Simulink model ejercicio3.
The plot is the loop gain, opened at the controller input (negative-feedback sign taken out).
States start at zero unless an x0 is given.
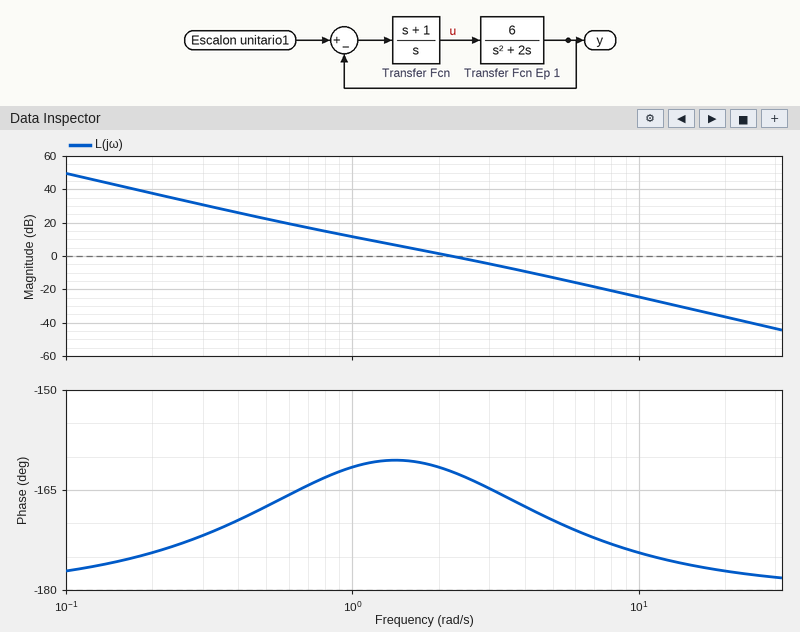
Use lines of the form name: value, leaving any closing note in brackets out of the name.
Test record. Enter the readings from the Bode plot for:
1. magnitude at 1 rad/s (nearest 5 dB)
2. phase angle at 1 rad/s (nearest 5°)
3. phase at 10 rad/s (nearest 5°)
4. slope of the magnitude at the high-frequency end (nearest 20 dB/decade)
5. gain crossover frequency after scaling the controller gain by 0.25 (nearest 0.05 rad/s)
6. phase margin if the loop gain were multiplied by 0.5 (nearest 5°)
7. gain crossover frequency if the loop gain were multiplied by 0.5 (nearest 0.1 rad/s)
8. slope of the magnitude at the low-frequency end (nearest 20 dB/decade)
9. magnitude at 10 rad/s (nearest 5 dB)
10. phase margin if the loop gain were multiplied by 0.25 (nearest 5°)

magnitude at 1 rad/s: 10 dB
phase angle at 1 rad/s: -160°
phase at 10 rad/s: -175°
slope of the magnitude at the high-frequency end: -40 dB/decade
gain crossover frequency after scaling the controller gain by 0.25: 0.95 rad/s
phase margin if the loop gain were multiplied by 0.5: 20°
gain crossover frequency if the loop gain were multiplied by 0.5: 1.5 rad/s
slope of the magnitude at the low-frequency end: -40 dB/decade
magnitude at 10 rad/s: -25 dB
phase margin if the loop gain were multiplied by 0.25: 20°
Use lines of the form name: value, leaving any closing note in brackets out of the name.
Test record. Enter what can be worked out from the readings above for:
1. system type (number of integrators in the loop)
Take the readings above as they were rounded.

system type: 2
